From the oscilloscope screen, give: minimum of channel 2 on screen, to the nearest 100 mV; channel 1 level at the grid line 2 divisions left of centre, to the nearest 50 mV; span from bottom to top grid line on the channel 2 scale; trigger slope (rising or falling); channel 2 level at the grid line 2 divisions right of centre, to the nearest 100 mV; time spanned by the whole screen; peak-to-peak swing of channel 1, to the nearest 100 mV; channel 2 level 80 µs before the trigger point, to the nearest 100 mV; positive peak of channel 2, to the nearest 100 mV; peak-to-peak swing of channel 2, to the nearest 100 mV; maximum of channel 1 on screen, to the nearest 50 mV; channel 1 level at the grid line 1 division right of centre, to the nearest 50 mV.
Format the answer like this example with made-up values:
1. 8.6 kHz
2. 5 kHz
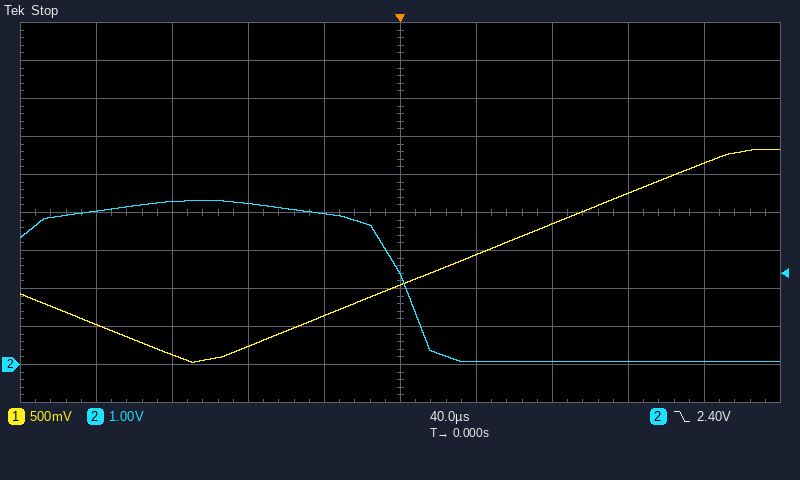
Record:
1. 100 mV
2. 250 mV
3. 10 V
4. falling
5. 100 mV
6. 400 µs
7. 2.80 V
8. 4.2 V
9. 4.3 V
10. 4.2 V
11. 2.85 V
12. 1.45 V
